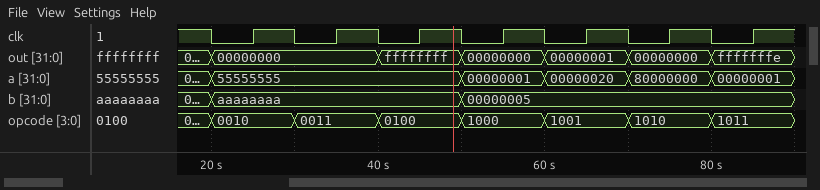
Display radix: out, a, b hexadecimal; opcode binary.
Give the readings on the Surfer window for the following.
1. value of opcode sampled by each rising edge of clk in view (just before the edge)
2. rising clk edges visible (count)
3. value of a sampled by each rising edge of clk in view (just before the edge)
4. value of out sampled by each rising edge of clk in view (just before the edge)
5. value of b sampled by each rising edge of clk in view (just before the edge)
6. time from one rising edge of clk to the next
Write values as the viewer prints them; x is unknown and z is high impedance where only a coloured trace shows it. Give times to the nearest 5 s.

0010, 0011, 0100, 1000, 1001, 1010, 1011
7
55555555, 55555555, 55555555, 00000001, 00000020, 80000000, 00000001
00000000, 00000000, ffffffff, 00000000, 00000001, 00000000, fffffffe
aaaaaaaa, aaaaaaaa, aaaaaaaa, 00000005, 00000005, 00000005, 00000005
10 s
